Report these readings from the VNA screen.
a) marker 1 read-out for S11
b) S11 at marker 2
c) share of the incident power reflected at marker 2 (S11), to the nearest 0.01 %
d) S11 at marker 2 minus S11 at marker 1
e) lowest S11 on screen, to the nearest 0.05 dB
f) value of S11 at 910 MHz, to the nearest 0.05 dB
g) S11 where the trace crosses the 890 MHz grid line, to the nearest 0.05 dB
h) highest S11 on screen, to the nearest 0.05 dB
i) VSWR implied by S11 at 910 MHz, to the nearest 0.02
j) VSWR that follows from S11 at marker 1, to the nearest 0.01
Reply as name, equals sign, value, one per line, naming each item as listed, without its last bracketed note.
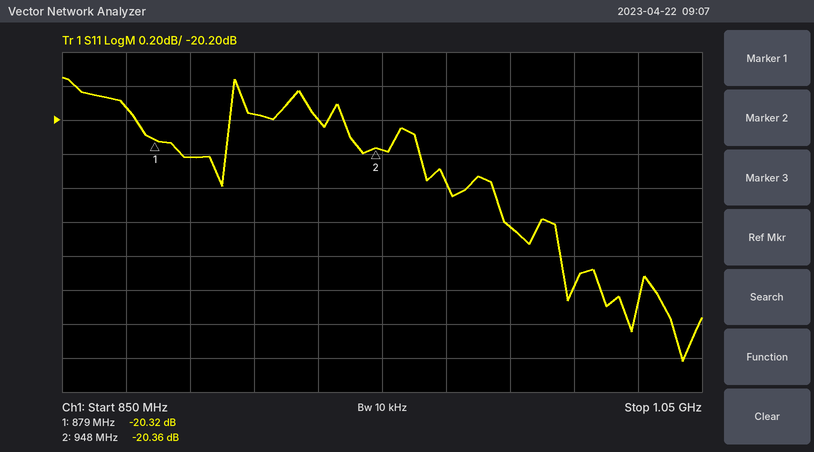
marker 1 read-out for S11 = -20.32 dB
S11 at marker 2 = -20.36 dB
share of the incident power reflected at marker 2 (S11), to the nearest 0.01 % = 0.92 %
S11 at marker 2 minus S11 at marker 1 = -0.04 dB
lowest S11 on screen, to the nearest 0.05 dB = -21.60 dB
value of S11 at 910 MHz, to the nearest 0.05 dB = -20.15 dB
S11 where the trace crosses the 890 MHz grid line, to the nearest 0.05 dB = -20.40 dB
highest S11 on screen, to the nearest 0.05 dB = -19.95 dB
VSWR implied by S11 at 910 MHz, to the nearest 0.02 = 1.22
VSWR that follows from S11 at marker 1, to the nearest 0.01 = 1.21
